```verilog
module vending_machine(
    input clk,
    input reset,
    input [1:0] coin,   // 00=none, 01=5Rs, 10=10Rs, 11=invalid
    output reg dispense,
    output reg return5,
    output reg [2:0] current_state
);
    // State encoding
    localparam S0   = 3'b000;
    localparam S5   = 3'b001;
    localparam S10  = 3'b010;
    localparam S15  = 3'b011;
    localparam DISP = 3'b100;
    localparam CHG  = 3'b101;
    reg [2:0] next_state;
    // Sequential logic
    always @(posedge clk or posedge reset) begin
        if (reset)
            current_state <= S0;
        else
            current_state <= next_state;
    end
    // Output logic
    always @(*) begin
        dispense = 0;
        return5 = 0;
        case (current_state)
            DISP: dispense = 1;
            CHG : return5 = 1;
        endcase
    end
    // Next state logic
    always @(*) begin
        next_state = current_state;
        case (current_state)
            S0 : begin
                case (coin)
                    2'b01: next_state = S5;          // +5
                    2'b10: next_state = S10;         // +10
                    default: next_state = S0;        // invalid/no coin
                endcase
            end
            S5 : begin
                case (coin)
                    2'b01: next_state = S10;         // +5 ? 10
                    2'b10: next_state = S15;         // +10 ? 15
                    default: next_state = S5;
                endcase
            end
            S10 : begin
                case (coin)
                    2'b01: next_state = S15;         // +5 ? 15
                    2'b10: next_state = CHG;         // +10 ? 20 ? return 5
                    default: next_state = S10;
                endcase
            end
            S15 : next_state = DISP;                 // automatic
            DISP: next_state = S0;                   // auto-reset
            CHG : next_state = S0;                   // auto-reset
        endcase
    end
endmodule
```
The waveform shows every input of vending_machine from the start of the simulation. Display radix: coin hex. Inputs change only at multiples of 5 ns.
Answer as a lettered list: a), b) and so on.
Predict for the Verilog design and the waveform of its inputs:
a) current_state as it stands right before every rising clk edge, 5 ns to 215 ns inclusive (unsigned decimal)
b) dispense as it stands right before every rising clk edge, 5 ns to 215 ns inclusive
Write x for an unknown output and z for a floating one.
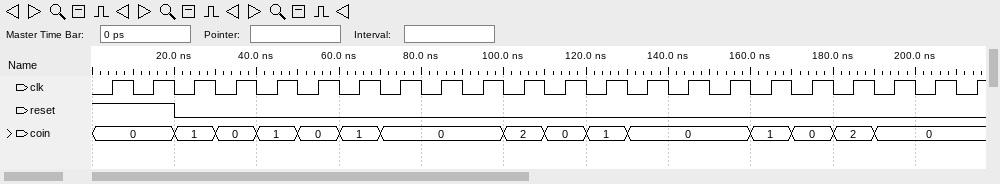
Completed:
a) 0, 0, 0, 1, 1, 2, 2, 3, 4, 0, 0, 2, 2, 3, 4, 0, 0, 1, 1, 3, 4, 0
b) 0 0 0 0 0 0 0 0 1 0 0 0 0 0 1 0 0 0 0 0 1 0
